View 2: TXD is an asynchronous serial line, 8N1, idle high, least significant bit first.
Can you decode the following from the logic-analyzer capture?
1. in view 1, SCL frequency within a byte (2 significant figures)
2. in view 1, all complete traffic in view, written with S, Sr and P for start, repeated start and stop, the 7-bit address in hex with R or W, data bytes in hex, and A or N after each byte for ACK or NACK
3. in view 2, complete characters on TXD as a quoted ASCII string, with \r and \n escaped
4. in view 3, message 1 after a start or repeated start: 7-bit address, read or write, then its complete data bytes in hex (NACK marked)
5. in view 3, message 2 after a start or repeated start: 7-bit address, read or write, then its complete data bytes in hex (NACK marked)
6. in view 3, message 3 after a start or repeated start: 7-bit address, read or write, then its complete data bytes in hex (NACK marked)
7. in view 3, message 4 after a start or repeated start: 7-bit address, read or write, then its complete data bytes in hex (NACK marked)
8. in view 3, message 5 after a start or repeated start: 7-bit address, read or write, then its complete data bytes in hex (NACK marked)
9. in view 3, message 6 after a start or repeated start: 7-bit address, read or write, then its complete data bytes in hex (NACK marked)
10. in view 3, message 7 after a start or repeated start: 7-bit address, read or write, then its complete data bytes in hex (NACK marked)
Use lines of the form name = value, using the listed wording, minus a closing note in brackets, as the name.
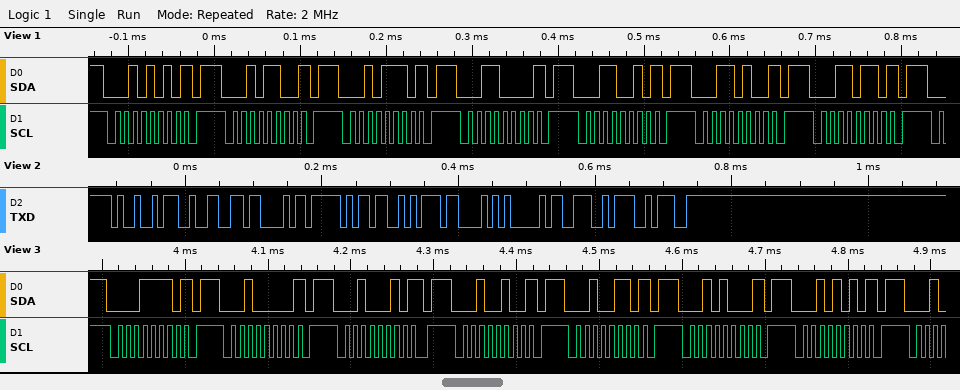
in view 1, SCL frequency within a byte = 100 kHz
in view 1, all complete traffic in view, written with S, Sr and P for start, repeated start and stop, the 7-bit address in hex with R or W, data bytes in hex, and A or N after each byte for ACK or NACK = S 15W N P S 16W N P S 17W N P S 18W N P S 19W N P S 1AW N P S 1BW N P
in view 2, complete characters on TXD as a quoted ASCII string, with \r and \n escaped = "I2C_SCAN:"
in view 3, message 1 after a start or repeated start: 7-bit address, read or write, then its complete data bytes in hex = 0x0F write NACK
in view 3, message 2 after a start or repeated start: 7-bit address, read or write, then its complete data bytes in hex = 0x10 write NACK
in view 3, message 3 after a start or repeated start: 7-bit address, read or write, then its complete data bytes in hex = 0x11 write NACK
in view 3, message 4 after a start or repeated start: 7-bit address, read or write, then its complete data bytes in hex = 0x12 write NACK
in view 3, message 5 after a start or repeated start: 7-bit address, read or write, then its complete data bytes in hex = 0x13 write NACK
in view 3, message 6 after a start or repeated start: 7-bit address, read or write, then its complete data bytes in hex = 0x14 write NACK
in view 3, message 7 after a start or repeated start: 7-bit address, read or write, then its complete data bytes in hex = 0x15 write NACK
